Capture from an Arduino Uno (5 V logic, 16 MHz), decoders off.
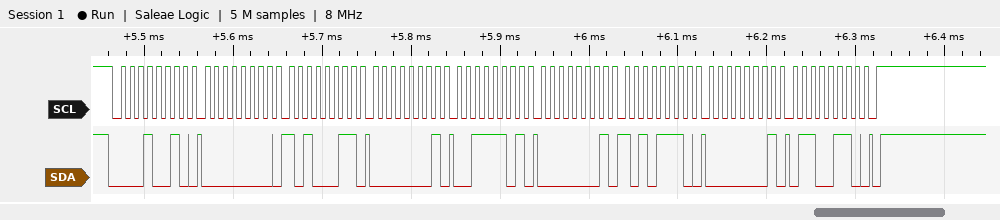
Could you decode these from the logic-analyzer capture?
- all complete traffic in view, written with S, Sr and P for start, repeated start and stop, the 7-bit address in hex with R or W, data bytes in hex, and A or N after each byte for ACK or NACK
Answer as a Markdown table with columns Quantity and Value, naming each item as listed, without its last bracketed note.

| Quantity | Value |
|---|---|
| all complete traffic in view, written with S, Sr and P for start, repeated start and stop, the 7-bit address in hex with R or W, data bytes in hex, and A or N after each byte for ACK or NACK | S 09W A 00 A A3 A 01 A 3D A 01 A AE A 01 A 66 A P |
